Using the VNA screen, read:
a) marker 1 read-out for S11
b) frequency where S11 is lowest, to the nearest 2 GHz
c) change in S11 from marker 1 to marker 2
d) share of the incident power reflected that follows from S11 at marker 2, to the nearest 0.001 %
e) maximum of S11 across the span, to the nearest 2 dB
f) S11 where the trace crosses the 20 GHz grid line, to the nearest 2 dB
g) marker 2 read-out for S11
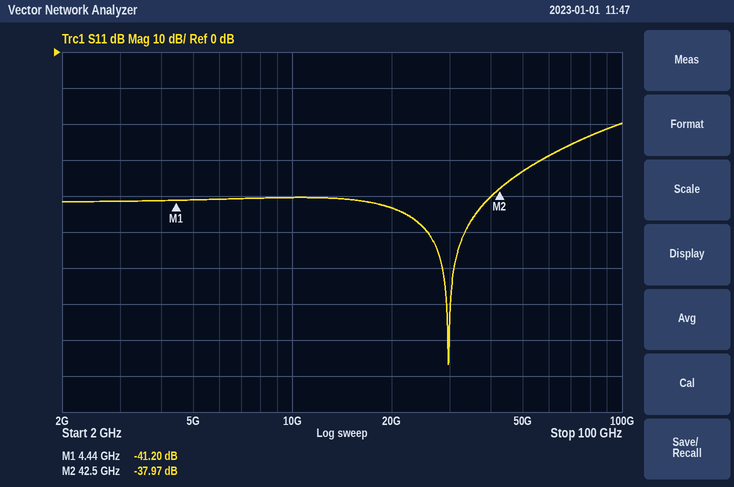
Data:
-41.20 dB
30 GHz
3.23 dB
0.016 %
-20 dB
-44 dB
-37.97 dB
